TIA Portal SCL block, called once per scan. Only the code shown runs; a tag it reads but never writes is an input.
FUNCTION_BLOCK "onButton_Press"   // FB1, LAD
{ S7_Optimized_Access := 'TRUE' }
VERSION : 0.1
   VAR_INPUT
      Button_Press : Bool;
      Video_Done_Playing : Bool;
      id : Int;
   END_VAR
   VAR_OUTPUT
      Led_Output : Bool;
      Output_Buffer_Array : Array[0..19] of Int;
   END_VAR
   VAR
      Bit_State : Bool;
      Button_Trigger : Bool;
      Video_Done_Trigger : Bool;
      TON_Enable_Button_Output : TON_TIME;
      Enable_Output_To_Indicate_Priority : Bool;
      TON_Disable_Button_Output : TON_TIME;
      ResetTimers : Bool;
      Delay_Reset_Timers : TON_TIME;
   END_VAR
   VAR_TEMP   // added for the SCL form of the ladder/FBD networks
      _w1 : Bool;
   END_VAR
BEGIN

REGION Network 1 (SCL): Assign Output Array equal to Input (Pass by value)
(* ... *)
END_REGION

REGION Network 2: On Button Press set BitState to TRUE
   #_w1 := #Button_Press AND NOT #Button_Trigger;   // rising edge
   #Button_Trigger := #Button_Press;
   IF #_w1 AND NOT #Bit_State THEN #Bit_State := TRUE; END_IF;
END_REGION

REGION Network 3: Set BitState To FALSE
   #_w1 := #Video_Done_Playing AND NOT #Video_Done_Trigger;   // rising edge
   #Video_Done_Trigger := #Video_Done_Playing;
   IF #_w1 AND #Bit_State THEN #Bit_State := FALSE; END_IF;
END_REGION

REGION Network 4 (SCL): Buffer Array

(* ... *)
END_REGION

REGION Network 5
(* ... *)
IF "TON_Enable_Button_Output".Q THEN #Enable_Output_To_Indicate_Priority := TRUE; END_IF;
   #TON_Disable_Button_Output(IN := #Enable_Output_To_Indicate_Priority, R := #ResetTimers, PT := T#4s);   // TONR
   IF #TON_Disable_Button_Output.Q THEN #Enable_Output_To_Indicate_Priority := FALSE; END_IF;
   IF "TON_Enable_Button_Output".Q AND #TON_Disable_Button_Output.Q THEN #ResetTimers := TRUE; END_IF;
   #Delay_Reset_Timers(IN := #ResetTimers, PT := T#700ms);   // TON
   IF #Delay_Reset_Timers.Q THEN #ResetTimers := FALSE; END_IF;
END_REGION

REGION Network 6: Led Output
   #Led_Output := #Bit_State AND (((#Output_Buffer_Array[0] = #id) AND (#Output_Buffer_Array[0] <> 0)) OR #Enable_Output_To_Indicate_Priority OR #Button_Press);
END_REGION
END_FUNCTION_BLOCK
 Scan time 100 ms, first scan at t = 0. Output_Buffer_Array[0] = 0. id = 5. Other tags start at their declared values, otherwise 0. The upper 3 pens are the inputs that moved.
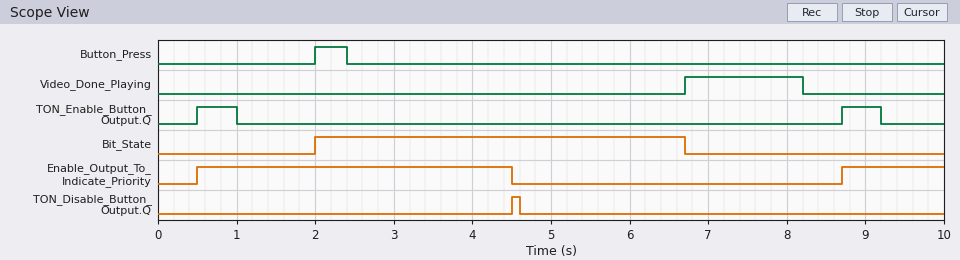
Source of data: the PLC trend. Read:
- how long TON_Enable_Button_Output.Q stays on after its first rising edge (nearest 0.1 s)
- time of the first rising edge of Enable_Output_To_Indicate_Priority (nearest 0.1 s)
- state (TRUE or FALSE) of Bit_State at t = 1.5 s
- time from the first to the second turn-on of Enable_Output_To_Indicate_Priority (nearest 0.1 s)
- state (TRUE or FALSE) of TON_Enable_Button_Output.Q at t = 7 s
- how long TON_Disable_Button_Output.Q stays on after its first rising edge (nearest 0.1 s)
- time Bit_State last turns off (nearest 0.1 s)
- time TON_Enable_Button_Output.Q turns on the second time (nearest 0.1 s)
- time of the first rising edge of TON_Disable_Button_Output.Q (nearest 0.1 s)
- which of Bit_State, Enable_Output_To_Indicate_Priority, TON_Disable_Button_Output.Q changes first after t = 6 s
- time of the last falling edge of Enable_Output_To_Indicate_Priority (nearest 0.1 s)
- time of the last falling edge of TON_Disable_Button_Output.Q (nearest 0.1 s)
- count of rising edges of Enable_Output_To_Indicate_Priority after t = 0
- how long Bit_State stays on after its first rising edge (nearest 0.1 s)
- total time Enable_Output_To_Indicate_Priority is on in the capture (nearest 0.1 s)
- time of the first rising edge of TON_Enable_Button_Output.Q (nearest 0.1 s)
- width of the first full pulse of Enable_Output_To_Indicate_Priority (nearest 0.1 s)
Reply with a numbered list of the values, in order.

1. 0.5 s
2. 0.5 s
3. FALSE
4. 8.2 s
5. FALSE
6. 0.1 s
7. 6.7 s
8. 8.7 s
9. 4.5 s
10. Bit_State
11. 4.5 s
12. 4.6 s
13. 2
14. 4.7 s
15. 5.3 s
16. 0.5 s
17. 4.0 s
